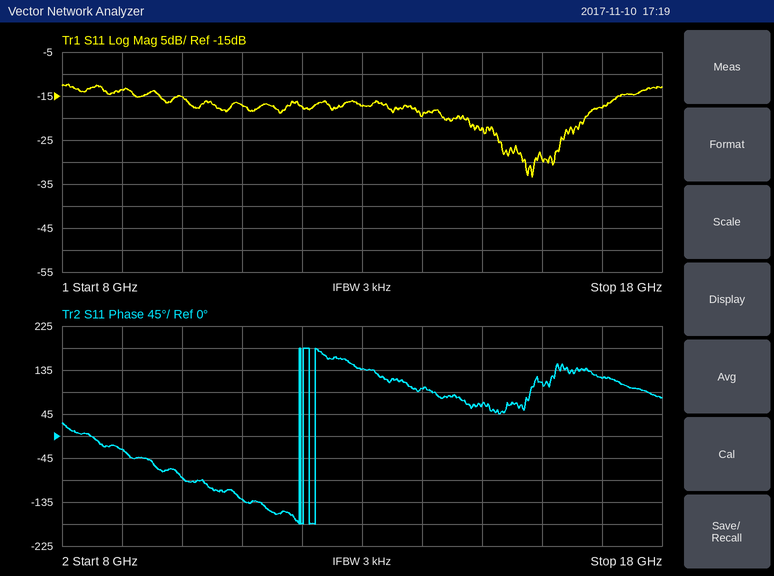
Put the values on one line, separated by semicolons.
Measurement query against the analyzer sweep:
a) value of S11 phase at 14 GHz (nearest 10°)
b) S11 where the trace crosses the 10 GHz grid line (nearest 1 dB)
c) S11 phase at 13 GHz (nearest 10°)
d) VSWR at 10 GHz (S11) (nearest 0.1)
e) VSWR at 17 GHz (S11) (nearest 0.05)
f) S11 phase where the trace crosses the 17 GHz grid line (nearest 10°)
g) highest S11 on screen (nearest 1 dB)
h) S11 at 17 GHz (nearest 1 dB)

100°; -15 dB; 140°; 1.4; 1.30; 120°; -12 dB; -18 dB
